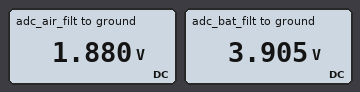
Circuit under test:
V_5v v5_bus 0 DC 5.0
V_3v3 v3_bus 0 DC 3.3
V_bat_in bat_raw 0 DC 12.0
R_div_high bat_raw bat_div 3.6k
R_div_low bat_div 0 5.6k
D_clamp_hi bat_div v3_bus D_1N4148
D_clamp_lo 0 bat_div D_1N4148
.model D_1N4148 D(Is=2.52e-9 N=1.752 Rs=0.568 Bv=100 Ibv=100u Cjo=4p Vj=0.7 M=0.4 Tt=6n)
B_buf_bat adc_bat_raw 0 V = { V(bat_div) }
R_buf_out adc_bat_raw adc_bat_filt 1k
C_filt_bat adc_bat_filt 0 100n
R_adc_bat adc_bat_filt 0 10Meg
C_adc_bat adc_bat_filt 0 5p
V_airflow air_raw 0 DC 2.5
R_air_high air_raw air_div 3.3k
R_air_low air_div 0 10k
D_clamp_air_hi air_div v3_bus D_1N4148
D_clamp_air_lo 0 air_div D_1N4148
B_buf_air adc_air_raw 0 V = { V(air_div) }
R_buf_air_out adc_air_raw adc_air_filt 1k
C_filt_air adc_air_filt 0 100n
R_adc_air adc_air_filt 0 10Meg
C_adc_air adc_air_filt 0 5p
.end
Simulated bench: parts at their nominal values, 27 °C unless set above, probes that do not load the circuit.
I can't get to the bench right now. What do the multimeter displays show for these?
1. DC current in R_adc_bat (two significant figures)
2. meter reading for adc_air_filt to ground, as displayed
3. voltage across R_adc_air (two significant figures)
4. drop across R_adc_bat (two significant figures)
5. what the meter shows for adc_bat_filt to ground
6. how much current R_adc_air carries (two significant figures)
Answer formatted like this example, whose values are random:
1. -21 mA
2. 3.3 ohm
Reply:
1. 390 nA
2. 1.880 V
3. 1.9 V
4. 3.9 V
5. 3.905 V
6. 190 nA
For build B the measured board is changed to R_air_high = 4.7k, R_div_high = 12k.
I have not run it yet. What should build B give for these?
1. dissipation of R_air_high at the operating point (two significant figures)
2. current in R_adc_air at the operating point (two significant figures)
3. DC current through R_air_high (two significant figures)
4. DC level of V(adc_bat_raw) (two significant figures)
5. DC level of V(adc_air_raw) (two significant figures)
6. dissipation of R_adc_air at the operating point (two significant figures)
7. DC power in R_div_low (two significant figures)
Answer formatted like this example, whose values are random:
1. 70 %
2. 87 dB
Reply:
1. 140 µW
2. 170 nA
3. 170 µA
4. 3.7 V
5. 1.7 V
6. 290 nW
7. 2.5 mW
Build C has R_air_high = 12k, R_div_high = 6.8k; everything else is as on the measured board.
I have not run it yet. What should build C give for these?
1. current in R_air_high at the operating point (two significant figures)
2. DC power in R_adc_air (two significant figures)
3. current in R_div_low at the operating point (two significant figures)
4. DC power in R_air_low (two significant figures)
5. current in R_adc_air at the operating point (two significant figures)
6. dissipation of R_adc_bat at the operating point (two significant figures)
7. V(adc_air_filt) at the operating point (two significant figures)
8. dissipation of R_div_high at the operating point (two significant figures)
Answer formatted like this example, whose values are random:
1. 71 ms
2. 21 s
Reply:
1. 110 µA
2. 130 nW
3. 690 µA
4. 130 µW
5. 110 nA
6. 1.5 µW
7. 1.1 V
8. 9.8 mW
